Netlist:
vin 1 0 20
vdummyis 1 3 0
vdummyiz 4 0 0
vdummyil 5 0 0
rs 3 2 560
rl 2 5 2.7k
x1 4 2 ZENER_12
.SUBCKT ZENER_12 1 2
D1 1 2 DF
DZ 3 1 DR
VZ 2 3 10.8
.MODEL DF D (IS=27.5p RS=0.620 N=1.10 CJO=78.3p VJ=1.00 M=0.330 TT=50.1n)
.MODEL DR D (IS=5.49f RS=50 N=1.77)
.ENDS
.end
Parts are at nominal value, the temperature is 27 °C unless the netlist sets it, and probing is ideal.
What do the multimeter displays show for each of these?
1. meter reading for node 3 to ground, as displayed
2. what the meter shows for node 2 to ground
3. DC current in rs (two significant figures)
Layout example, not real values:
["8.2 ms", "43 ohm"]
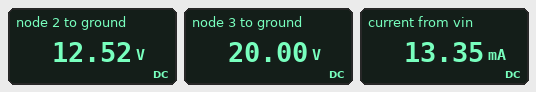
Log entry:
["20.00 V", "12.52 V", "13 mA"]
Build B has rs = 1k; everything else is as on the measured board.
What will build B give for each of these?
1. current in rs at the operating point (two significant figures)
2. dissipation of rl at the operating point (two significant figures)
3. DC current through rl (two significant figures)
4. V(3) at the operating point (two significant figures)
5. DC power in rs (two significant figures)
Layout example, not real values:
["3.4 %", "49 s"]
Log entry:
["7.8 mA", "55 mW", "4.5 mA", "20 V", "61 mW"]
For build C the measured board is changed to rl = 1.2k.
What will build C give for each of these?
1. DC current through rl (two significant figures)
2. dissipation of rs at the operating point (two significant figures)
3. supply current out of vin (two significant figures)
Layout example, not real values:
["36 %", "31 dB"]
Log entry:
["10 mA", "110 mW", "14 mA"]
